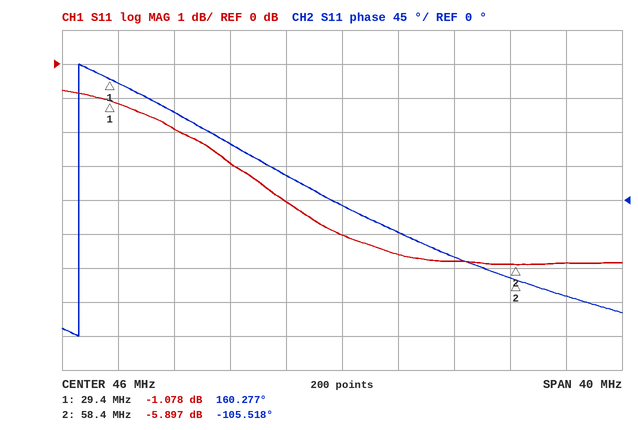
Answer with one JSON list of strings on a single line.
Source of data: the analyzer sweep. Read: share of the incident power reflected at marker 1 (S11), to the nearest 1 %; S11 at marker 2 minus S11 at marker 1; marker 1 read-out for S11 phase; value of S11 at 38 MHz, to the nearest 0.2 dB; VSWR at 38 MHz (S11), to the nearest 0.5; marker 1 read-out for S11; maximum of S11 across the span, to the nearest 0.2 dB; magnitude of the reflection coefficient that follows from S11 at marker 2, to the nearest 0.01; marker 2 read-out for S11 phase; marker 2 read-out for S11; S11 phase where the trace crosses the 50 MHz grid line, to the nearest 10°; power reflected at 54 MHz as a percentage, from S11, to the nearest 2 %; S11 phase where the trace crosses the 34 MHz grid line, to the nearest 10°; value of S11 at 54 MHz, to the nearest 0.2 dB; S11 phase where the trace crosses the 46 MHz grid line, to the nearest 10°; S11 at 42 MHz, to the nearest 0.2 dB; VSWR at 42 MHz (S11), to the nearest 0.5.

["78 %", "-4.819 dB", "160.277°", "-3.0 dB", "6.0", "-1.078 dB", "-0.8 dB", "0.51", "-105.518°", "-5.897 dB", "-40°", "26 %", "120°", "-5.8 dB", "-10°", "-4.0 dB", "4.5"]
